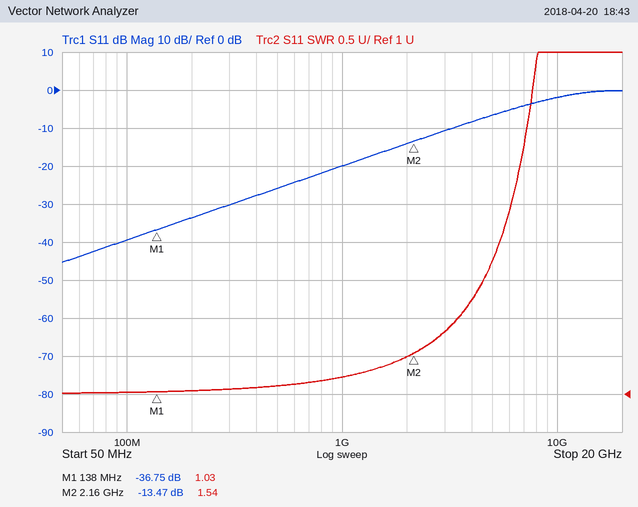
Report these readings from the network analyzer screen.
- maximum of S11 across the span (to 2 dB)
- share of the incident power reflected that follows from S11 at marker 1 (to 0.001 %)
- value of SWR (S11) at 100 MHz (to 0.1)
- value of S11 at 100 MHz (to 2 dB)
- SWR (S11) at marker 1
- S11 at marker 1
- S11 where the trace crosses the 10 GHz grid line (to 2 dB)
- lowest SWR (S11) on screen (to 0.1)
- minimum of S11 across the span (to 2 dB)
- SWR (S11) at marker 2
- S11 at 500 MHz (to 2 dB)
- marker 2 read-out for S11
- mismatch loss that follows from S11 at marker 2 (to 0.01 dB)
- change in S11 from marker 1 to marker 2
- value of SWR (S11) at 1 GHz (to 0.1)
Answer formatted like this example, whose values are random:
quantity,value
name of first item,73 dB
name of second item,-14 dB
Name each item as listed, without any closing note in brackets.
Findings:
quantity,value
maximum of S11 across the span,0 dB
share of the incident power reflected that follows from S11 at marker 1,0.021 %
value of SWR (S11) at 100 MHz,1.0
value of S11 at 100 MHz,-40 dB
SWR (S11) at marker 1,1.03
S11 at marker 1,-36.75 dB
S11 where the trace crosses the 10 GHz grid line,-2 dB
lowest SWR (S11) on screen,1.0
minimum of S11 across the span,-46 dB
SWR (S11) at marker 2,1.54
S11 at 500 MHz,-26 dB
marker 2 read-out for S11,-13.47 dB
mismatch loss that follows from S11 at marker 2,0.20 dB
change in S11 from marker 1 to marker 2,23.28 dB
value of SWR (S11) at 1 GHz,1.2
